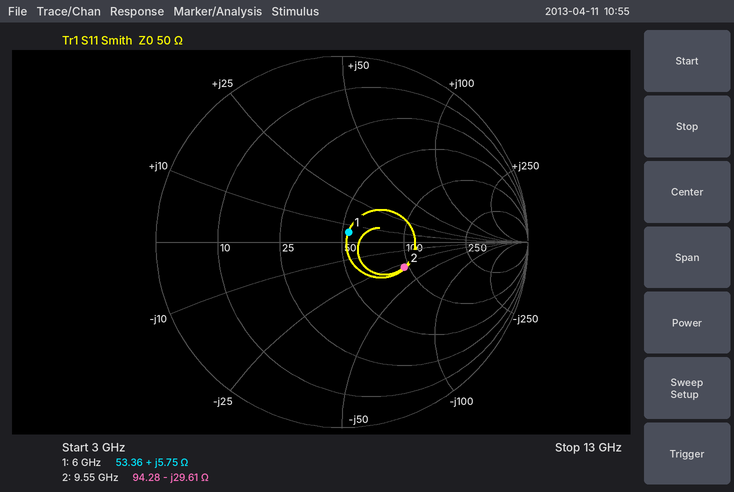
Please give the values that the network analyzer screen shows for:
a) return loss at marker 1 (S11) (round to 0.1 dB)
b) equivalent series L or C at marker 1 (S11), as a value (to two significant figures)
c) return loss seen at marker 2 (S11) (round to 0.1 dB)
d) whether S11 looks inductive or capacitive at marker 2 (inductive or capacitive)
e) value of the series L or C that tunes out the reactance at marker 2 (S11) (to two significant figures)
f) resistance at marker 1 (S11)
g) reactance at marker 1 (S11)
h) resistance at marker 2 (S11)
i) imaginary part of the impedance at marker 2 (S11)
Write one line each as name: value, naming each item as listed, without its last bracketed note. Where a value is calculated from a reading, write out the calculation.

return loss at marker 1 (S11): 23.8 dB
equivalent series L or C at marker 1 (S11), as a value: L = 5.75 Ω/(2π × 6 GHz) ≈ 153 pH, so 150 pH to two significant figures
return loss seen at marker 2 (S11): 8.8 dB
whether S11 looks inductive or capacitive at marker 2: capacitive
value of the series L or C that tunes out the reactance at marker 2 (S11): L = 29.61 Ω/(2π × 9.55 GHz) ≈ 493 pH, so 490 pH to two significant figures
resistance at marker 1: 53.36 Ω
reactance at marker 1: +5.75 Ω
resistance at marker 2: 94.28 Ω
imaginary part of the impedance at marker 2: -29.61 Ω
